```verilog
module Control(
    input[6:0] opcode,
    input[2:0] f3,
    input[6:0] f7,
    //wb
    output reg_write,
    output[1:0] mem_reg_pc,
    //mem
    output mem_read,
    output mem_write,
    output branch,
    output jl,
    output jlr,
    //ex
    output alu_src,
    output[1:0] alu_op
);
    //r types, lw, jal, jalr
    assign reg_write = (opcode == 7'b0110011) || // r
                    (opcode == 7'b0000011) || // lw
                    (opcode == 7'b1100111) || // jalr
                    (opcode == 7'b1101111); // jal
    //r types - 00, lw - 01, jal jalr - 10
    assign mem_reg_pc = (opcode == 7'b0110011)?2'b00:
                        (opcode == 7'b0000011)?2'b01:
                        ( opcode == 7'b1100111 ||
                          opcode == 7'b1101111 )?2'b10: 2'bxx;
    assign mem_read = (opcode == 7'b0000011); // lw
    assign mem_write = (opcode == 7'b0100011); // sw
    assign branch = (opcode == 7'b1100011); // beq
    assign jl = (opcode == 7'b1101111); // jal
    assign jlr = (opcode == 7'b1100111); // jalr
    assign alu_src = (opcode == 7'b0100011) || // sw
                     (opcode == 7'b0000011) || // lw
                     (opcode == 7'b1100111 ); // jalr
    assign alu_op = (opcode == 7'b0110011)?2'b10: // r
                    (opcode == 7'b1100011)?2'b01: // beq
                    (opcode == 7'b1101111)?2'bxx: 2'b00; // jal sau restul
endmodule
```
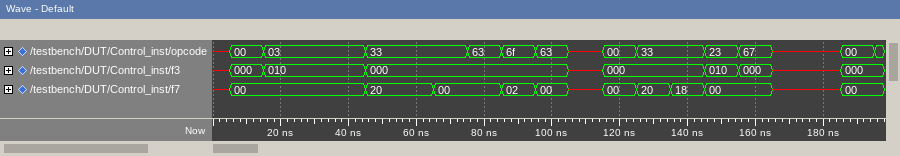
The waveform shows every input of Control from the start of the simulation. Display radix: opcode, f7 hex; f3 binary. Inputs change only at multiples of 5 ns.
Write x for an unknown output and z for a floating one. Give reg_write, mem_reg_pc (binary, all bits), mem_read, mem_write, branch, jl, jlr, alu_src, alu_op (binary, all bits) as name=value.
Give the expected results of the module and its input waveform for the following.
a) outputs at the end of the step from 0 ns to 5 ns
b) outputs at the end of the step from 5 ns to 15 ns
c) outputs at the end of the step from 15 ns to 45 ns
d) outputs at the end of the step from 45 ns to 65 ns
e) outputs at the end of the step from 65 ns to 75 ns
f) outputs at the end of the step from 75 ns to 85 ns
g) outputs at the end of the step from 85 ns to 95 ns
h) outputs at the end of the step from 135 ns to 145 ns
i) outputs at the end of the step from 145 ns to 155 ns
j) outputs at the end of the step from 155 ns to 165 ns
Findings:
reg_write=x, mem_reg_pc=x, mem_read=x, mem_write=x, branch=x, jl=x, jlr=x, alu_src=x, alu_op=x
reg_write=0, mem_reg_pc=x, mem_read=0, mem_write=0, branch=0, jl=0, jlr=0, alu_src=0, alu_op=00
reg_write=1, mem_reg_pc=01, mem_read=1, mem_write=0, branch=0, jl=0, jlr=0, alu_src=1, alu_op=00
reg_write=1, mem_reg_pc=00, mem_read=0, mem_write=0, branch=0, jl=0, jlr=0, alu_src=0, alu_op=10
reg_write=1, mem_reg_pc=00, mem_read=0, mem_write=0, branch=0, jl=0, jlr=0, alu_src=0, alu_op=10
reg_write=0, mem_reg_pc=x, mem_read=0, mem_write=0, branch=1, jl=0, jlr=0, alu_src=0, alu_op=01
reg_write=1, mem_reg_pc=10, mem_read=0, mem_write=0, branch=0, jl=1, jlr=0, alu_src=0, alu_op=x
reg_write=1, mem_reg_pc=00, mem_read=0, mem_write=0, branch=0, jl=0, jlr=0, alu_src=0, alu_op=10
reg_write=0, mem_reg_pc=x, mem_read=0, mem_write=1, branch=0, jl=0, jlr=0, alu_src=1, alu_op=00
reg_write=1, mem_reg_pc=10, mem_read=0, mem_write=0, branch=0, jl=0, jlr=1, alu_src=1, alu_op=00
